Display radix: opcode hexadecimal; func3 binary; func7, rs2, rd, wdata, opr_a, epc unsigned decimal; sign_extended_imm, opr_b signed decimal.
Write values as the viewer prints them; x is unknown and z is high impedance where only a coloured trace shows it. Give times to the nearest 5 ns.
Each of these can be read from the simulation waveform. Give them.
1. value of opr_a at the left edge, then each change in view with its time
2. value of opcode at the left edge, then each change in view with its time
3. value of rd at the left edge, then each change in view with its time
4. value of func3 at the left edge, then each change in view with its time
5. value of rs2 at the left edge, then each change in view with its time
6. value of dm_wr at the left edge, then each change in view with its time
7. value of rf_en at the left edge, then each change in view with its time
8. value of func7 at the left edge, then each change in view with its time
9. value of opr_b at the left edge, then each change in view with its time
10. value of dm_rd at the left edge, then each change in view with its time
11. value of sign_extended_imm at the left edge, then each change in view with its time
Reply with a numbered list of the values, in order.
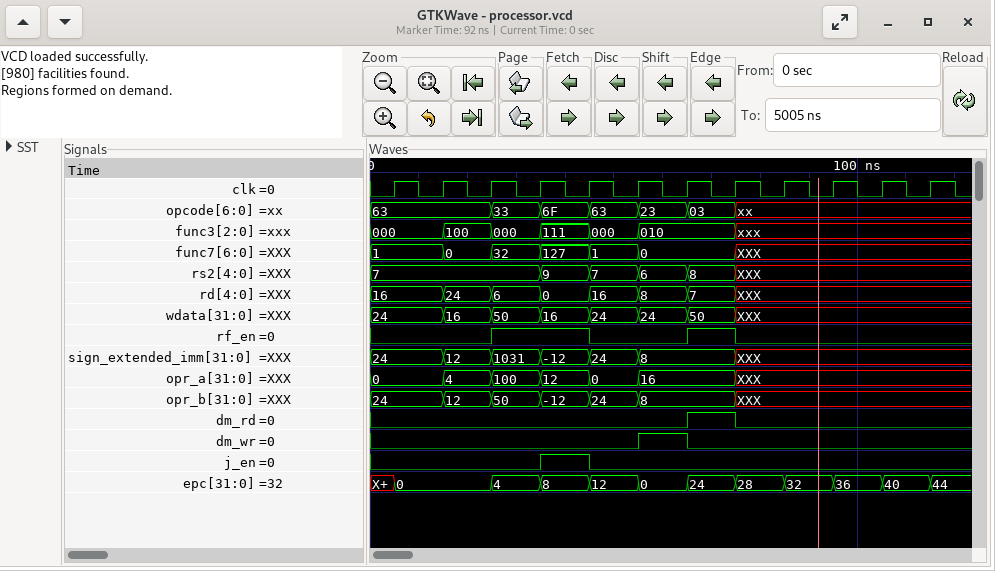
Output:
1. 0, 4 at 15 ns, 100 at 25 ns, 12 at 35 ns, 0 at 45 ns, 16 at 55 ns, XXX at 75 ns
2. 63, 33 at 25 ns, 6F at 35 ns, 63 at 45 ns, 23 at 55 ns, 03 at 65 ns, xx at 75 ns
3. 16, 24 at 15 ns, 6 at 25 ns, 0 at 35 ns, 16 at 45 ns, 8 at 55 ns, 7 at 65 ns, XXX at 75 ns
4. 000, 100 at 15 ns, 000 at 25 ns, 111 at 35 ns, 000 at 45 ns, 010 at 55 ns, xxx at 75 ns
5. 7, 9 at 35 ns, 7 at 45 ns, 6 at 55 ns, 8 at 65 ns, XXX at 75 ns
6. 0, 1 at 55 ns, 0 at 65 ns
7. 0, 1 at 25 ns, 0 at 45 ns, 1 at 65 ns, 0 at 75 ns
8. 1, 0 at 15 ns, 32 at 25 ns, 127 at 35 ns, 1 at 45 ns, 0 at 55 ns, XXX at 75 ns
9. 24, 12 at 15 ns, 50 at 25 ns, -12 at 35 ns, 24 at 45 ns, 8 at 55 ns, XXX at 75 ns
10. 0, 1 at 65 ns, 0 at 75 ns
11. 24, 12 at 15 ns, 1031 at 25 ns, -12 at 35 ns, 24 at 45 ns, 8 at 55 ns, XXX at 75 ns
